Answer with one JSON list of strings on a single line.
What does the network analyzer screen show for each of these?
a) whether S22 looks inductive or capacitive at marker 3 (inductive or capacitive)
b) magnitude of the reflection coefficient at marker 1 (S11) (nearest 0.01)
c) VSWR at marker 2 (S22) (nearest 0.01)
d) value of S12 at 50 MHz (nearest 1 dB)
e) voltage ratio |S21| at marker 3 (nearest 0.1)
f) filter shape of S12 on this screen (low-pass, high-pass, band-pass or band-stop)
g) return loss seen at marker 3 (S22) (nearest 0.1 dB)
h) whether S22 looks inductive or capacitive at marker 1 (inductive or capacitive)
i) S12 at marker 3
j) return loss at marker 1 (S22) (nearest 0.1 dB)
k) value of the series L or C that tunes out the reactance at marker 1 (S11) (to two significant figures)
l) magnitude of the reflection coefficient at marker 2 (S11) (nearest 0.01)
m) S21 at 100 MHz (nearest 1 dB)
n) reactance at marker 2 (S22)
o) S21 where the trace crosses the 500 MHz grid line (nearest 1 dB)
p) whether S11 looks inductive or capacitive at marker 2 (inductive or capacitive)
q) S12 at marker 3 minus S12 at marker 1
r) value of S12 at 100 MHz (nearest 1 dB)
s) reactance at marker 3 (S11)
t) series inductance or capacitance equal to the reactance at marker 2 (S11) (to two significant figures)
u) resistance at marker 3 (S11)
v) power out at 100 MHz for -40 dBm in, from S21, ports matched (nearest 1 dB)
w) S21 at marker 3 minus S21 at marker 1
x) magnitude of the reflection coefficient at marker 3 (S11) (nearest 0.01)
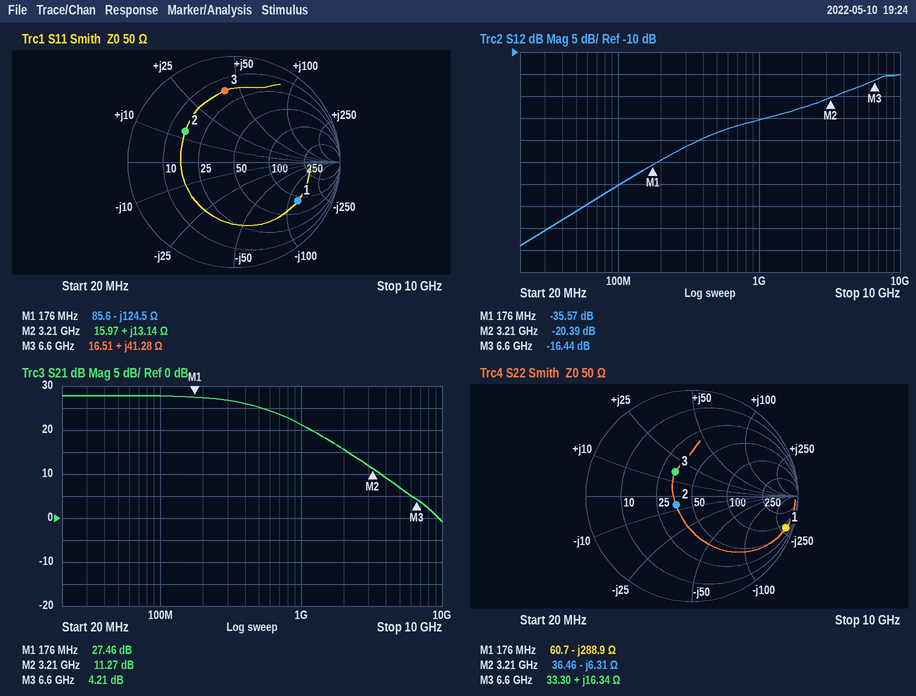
["inductive", "0.70", "1.42", "-46 dB", "1.6", "high-pass", "11.2 dB", "capacitive", "-16.44 dB", "0.6 dB", "110 nH", "0.54", "28 dB", "-6.31 Ω", "25 dB", "inductive", "19.13 dB", "-40 dB", "+41.28 Ω", "650 pH", "16.51 Ω", "-12 dBm", "-23.25 dB", "0.68"]
